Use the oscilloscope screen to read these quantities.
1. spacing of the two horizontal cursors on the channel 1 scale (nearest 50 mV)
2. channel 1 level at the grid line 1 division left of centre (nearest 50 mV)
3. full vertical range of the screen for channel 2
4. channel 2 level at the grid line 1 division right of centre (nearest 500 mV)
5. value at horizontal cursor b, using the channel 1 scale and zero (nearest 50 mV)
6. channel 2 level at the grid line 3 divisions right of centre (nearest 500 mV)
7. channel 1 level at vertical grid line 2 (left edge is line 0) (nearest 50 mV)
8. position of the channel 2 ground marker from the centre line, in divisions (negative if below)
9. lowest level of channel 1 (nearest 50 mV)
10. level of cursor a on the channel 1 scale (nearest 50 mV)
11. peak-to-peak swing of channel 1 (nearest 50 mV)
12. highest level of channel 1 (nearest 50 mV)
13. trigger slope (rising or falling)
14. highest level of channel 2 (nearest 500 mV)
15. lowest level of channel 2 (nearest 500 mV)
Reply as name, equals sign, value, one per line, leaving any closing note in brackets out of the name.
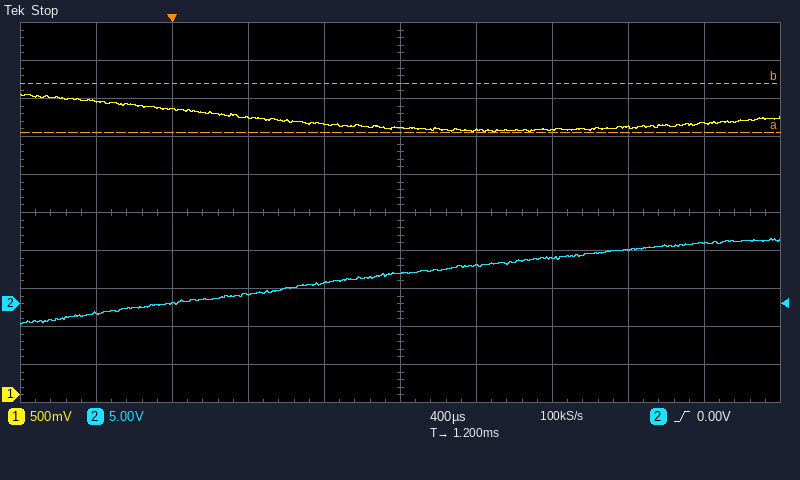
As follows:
spacing of the two horizontal cursors on the channel 1 scale = 650 mV
channel 1 level at the grid line 1 division left of centre = 3.55 V
full vertical range of the screen for channel 2 = 50 V
channel 2 level at the grid line 1 division right of centre = 5.0 V
value at horizontal cursor b, using the channel 1 scale and zero = 4.10 V
channel 2 level at the grid line 3 divisions right of centre = 7.0 V
channel 1 level at vertical grid line 2 (left edge is line 0) = 3.75 V
position of the channel 2 ground marker from the centre line, in divisions = -2.4 div
lowest level of channel 1 = 3.45 V
level of cursor a on the channel 1 scale = 3.45 V
peak-to-peak swing of channel 1 = 500 mV
highest level of channel 1 = 3.95 V
trigger slope = rising
highest level of channel 2 = 8.5 V
lowest level of channel 2 = -2.5 V
